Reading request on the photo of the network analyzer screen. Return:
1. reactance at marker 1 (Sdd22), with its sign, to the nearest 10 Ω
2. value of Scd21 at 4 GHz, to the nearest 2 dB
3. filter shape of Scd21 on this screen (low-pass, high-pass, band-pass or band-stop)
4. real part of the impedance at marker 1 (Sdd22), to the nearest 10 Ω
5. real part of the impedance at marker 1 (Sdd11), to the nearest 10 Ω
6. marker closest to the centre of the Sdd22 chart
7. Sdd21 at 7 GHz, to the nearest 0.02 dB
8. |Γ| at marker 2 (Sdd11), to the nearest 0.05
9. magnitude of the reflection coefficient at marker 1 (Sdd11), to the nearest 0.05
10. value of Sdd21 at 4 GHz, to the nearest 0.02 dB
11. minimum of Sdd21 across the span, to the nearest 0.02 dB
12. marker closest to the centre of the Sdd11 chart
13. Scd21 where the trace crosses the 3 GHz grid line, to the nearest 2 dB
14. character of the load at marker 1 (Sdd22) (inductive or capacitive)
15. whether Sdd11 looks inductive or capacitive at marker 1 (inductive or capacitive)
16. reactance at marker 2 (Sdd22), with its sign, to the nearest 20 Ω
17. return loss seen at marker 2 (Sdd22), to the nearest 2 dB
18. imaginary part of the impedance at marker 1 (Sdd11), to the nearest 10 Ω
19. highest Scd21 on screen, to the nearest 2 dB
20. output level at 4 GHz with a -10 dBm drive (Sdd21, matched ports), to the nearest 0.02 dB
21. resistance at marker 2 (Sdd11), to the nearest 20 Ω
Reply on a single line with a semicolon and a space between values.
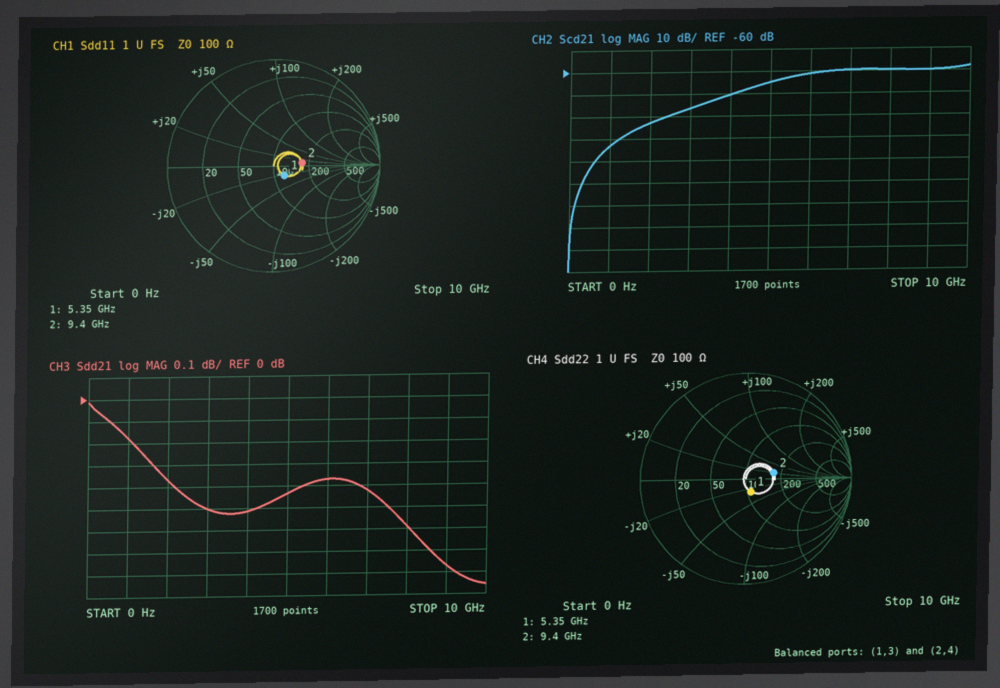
-30 Ω; -70 dB; high-pass; 110 Ω; 120 Ω; marker 1; -0.42 dB; 0.25; 0.15; -0.52 dB; -0.86 dB; marker 1; -76 dB; capacitive; capacitive; +20 Ω; 12 dB; -20 Ω; -58 dB; -10.52 dBm; 180 Ω
